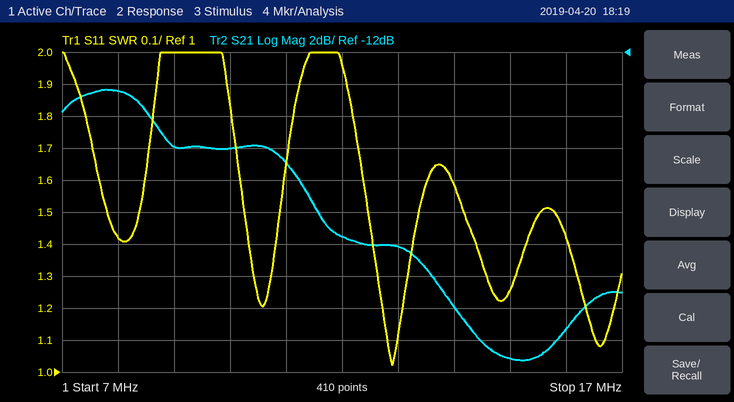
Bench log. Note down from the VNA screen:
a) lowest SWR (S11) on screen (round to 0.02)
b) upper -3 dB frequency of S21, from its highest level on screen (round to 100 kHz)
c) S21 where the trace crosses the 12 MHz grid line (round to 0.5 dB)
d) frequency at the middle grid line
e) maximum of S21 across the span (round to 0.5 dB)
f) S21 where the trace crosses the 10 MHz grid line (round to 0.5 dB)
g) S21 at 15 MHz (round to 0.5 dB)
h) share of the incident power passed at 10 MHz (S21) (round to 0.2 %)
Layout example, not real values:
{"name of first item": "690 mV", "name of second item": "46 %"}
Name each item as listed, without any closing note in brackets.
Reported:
{"lowest SWR (S11) on screen": "1.02", "upper -3 dB frequency of S21, from its highest level on screen": "8.8 MHz", "S21 where the trace crosses the 12 MHz grid line": "-23.5 dB", "frequency at the middle grid line": "12 MHz", "maximum of S21 across the span": "-14.5 dB", "S21 where the trace crosses the 10 MHz grid line": "-18.0 dB", "S21 at 15 MHz": "-31.0 dB", "share of the incident power passed at 10 MHz (S21)": "1.6 %"}
